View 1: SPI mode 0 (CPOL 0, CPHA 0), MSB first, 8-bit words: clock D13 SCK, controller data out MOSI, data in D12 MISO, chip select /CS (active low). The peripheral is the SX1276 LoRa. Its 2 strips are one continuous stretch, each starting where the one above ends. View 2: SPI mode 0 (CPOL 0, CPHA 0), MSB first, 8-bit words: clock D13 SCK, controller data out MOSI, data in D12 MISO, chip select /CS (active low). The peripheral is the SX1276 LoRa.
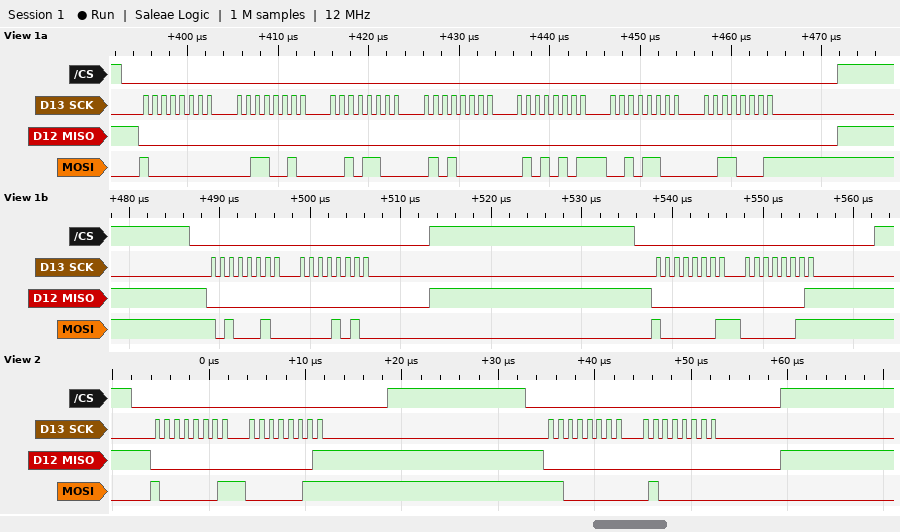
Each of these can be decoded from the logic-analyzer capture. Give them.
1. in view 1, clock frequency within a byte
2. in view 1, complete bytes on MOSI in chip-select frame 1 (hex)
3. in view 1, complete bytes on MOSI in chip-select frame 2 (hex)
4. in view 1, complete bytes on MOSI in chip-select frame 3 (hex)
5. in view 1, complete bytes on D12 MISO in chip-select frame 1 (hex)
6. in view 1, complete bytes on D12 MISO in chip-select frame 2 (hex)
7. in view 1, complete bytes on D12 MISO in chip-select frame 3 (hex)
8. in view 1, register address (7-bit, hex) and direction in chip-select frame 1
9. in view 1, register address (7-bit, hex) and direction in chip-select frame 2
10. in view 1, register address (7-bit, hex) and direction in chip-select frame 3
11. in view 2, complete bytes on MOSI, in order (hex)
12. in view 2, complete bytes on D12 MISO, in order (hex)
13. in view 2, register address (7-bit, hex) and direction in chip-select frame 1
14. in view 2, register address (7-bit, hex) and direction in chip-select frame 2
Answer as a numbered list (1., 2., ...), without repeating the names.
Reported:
1. 1 MHz
2. 0x80 0x32 0x2C 0x50 0x55 0x2C 0x31
3. 0xA2 0x0A
4. 0x81 0x03
5. 0x00 0x00 0x00 0x00 0x00 0x00 0x00
6. 0x00 0x00
7. 0x00 0x01
8. 0x00 write
9. 0x22 write
10. 0x01 write
11. 0x81 0x03 0xC0 0x40
12. 0x00 0x01 0x00 0x00
13. 0x01 write
14. 0x40 write
